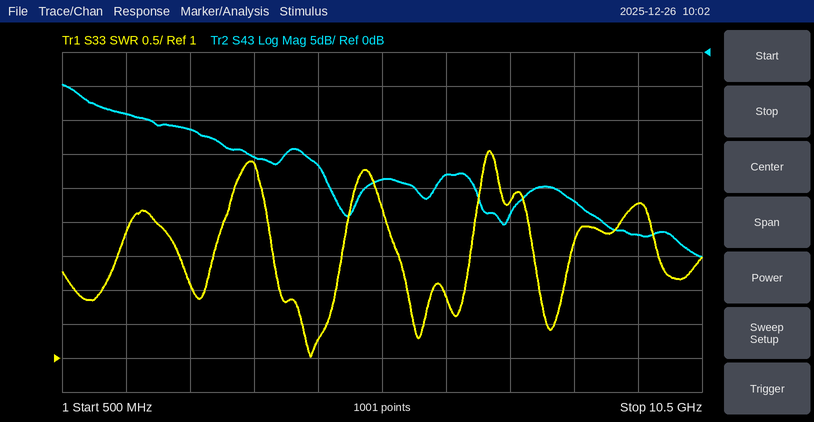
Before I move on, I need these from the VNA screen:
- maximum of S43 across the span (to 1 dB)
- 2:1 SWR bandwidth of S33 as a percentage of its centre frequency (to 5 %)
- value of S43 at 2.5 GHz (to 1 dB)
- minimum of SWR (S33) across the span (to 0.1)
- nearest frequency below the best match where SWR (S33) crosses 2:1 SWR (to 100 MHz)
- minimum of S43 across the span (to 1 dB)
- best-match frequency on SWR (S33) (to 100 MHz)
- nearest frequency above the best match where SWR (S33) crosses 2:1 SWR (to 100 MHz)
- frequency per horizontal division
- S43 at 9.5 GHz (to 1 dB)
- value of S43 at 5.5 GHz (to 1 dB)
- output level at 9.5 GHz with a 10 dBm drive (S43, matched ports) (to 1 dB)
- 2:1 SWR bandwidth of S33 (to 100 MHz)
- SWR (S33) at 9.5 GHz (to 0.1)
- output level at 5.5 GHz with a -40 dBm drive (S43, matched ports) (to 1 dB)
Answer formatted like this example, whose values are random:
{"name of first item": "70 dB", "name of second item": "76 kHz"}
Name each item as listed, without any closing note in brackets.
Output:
{"maximum of S43 across the span": "-5 dB", "2:1 SWR bandwidth of S33 as a percentage of its centre frequency": "20 %", "value of S43 at 2.5 GHz": "-11 dB", "minimum of SWR (S33) across the span": "1.0", "nearest frequency below the best match where SWR (S33) crosses 2:1 SWR": "3.9 GHz", "minimum of S43 across the span": "-30 dB", "best-match frequency on SWR (S33)": "4.4 GHz", "nearest frequency above the best match where SWR (S33) crosses 2:1 SWR": "4.8 GHz", "frequency per horizontal division": "1 GHz", "S43 at 9.5 GHz": "-27 dB", "value of S43 at 5.5 GHz": "-19 dB", "output level at 9.5 GHz with a 10 dBm drive (S43, matched ports)": "-17 dBm", "2:1 SWR bandwidth of S33": "900 MHz", "SWR (S33) at 9.5 GHz": "3.3", "output level at 5.5 GHz with a -40 dBm drive (S43, matched ports)": "-59 dBm"}
